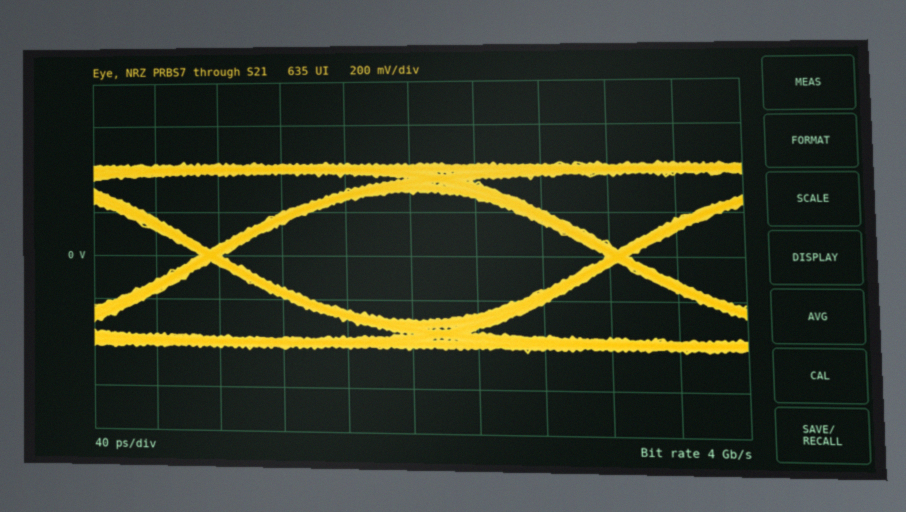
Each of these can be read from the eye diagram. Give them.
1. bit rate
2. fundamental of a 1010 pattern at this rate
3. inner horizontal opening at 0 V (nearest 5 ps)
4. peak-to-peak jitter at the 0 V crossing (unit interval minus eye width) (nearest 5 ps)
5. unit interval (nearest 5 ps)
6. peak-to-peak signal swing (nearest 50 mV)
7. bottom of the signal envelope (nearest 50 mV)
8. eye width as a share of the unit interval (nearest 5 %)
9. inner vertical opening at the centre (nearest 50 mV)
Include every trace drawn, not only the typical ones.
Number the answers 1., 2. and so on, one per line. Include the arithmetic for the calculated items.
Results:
1. 4 Gb/s
2. 2 GHz
3. 235 ps
4. 15 ps
5. 250 ps
6. 850 mV
7. -450 mV
8. 235 ps / 250 ps ≈ 94.0 %, so 95 % to the nearest 5 %
9. 600 mV
